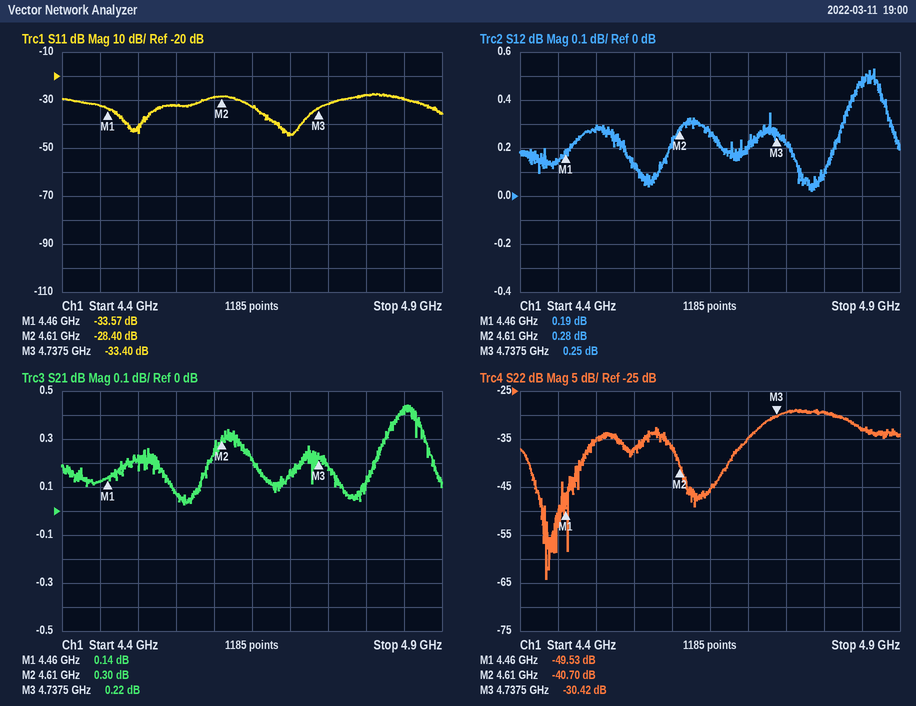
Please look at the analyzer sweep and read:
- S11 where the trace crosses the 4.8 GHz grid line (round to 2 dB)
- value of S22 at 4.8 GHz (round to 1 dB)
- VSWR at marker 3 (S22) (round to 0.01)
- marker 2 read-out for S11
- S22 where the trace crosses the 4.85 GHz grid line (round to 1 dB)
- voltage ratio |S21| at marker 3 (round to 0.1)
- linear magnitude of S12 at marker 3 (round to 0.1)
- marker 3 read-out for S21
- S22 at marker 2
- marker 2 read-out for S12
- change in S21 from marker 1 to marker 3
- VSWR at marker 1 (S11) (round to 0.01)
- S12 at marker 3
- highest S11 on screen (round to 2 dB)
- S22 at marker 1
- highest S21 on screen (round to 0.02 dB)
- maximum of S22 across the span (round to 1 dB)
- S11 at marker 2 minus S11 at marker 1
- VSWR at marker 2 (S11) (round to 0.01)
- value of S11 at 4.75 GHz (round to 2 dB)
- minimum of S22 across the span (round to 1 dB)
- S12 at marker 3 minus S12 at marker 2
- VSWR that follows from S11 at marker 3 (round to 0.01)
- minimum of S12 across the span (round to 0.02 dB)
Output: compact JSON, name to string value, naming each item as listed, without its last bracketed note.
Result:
{"S11 where the trace crosses the 4.8 GHz grid line": "-28 dB", "value of S22 at 4.8 GHz": "-29 dB", "VSWR at marker 3 (S22)": "1.06", "marker 2 read-out for S11": "-28.40 dB", "S22 where the trace crosses the 4.85 GHz grid line": "-33 dB", "voltage ratio |S21| at marker 3": "1.0", "linear magnitude of S12 at marker 3": "1.0", "marker 3 read-out for S21": "0.22 dB", "S22 at marker 2": "-40.70 dB", "marker 2 read-out for S12": "0.28 dB", "change in S21 from marker 1 to marker 3": "0.08 dB", "VSWR at marker 1 (S11)": "1.04", "S12 at marker 3": "0.25 dB", "highest S11 on screen": "-28 dB", "S22 at marker 1": "-49.53 dB", "highest S21 on screen": "0.44 dB", "maximum of S22 across the span": "-29 dB", "S11 at marker 2 minus S11 at marker 1": "5.17 dB", "VSWR at marker 2 (S11)": "1.08", "value of S11 at 4.75 GHz": "-32 dB", "minimum of S22 across the span": "-64 dB", "S12 at marker 3 minus S12 at marker 2": "-0.03 dB", "VSWR that follows from S11 at marker 3": "1.04", "minimum of S12 across the span": "0.02 dB"}
